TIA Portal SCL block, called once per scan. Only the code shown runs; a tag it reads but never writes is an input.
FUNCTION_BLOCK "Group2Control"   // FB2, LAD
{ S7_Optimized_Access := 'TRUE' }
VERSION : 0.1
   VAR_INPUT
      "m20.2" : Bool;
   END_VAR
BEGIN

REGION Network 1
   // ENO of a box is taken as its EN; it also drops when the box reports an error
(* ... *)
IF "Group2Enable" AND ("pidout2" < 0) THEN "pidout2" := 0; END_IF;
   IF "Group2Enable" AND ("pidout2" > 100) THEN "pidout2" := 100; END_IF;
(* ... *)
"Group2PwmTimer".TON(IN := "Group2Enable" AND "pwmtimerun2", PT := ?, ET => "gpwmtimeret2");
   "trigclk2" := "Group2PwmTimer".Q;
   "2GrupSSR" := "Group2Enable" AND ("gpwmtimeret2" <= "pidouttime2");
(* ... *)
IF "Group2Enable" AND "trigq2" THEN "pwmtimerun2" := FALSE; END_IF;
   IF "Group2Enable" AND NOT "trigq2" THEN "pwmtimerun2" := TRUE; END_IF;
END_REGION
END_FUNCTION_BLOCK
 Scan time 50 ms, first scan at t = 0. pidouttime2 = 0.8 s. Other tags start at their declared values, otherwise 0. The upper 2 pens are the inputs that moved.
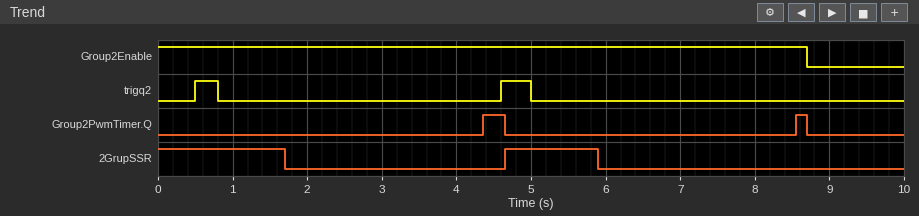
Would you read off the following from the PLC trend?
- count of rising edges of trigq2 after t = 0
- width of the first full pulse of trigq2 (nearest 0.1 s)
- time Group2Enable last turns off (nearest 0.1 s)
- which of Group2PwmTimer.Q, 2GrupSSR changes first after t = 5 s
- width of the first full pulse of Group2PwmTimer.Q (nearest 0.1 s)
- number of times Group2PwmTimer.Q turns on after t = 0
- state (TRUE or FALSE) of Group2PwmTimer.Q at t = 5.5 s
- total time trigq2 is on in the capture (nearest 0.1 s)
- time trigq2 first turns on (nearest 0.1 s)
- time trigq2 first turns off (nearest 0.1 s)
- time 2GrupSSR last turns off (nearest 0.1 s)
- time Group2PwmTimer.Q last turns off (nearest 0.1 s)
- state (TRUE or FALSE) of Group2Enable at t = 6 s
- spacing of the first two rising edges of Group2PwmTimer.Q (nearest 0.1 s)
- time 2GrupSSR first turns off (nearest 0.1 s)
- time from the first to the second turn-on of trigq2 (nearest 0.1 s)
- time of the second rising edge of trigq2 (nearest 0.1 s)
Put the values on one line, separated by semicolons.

2; 0.3 s; 8.7 s; 2GrupSSR; 0.3 s; 2; FALSE; 0.7 s; 0.5 s; 0.8 s; 5.9 s; 8.7 s; TRUE; 4.2 s; 1.7 s; 4.1 s; 4.6 s
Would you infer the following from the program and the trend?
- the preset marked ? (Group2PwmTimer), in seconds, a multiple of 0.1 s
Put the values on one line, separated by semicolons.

3.5 s
